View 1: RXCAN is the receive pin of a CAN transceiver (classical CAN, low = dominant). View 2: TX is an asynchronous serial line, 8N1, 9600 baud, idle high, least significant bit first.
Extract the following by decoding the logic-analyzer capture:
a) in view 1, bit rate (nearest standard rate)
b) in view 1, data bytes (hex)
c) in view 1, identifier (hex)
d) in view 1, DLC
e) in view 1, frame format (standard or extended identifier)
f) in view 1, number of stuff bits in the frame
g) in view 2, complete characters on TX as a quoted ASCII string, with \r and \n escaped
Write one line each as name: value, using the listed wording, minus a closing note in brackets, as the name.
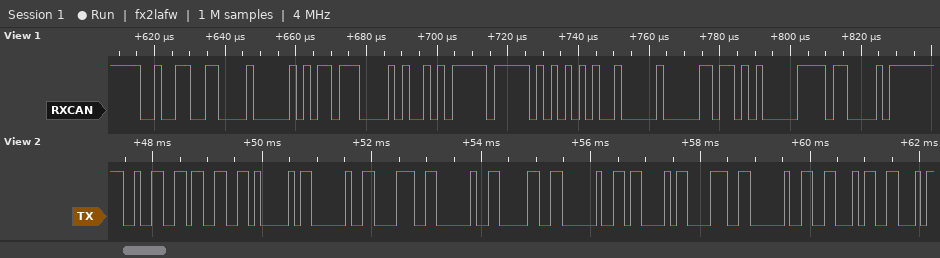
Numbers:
in view 1, bit rate: 500 kbit/s
in view 1, data bytes: 16 E1 4A FF EA A4 00 B5
in view 1, identifier: 0x266
in view 1, DLC: 8
in view 1, frame format: standard
in view 1, number of stuff bits in the frame: 6
in view 2, complete characters on TX as a quoted ASCII string, with \r and \n escaped: "23A 8 0 C8 FF"
